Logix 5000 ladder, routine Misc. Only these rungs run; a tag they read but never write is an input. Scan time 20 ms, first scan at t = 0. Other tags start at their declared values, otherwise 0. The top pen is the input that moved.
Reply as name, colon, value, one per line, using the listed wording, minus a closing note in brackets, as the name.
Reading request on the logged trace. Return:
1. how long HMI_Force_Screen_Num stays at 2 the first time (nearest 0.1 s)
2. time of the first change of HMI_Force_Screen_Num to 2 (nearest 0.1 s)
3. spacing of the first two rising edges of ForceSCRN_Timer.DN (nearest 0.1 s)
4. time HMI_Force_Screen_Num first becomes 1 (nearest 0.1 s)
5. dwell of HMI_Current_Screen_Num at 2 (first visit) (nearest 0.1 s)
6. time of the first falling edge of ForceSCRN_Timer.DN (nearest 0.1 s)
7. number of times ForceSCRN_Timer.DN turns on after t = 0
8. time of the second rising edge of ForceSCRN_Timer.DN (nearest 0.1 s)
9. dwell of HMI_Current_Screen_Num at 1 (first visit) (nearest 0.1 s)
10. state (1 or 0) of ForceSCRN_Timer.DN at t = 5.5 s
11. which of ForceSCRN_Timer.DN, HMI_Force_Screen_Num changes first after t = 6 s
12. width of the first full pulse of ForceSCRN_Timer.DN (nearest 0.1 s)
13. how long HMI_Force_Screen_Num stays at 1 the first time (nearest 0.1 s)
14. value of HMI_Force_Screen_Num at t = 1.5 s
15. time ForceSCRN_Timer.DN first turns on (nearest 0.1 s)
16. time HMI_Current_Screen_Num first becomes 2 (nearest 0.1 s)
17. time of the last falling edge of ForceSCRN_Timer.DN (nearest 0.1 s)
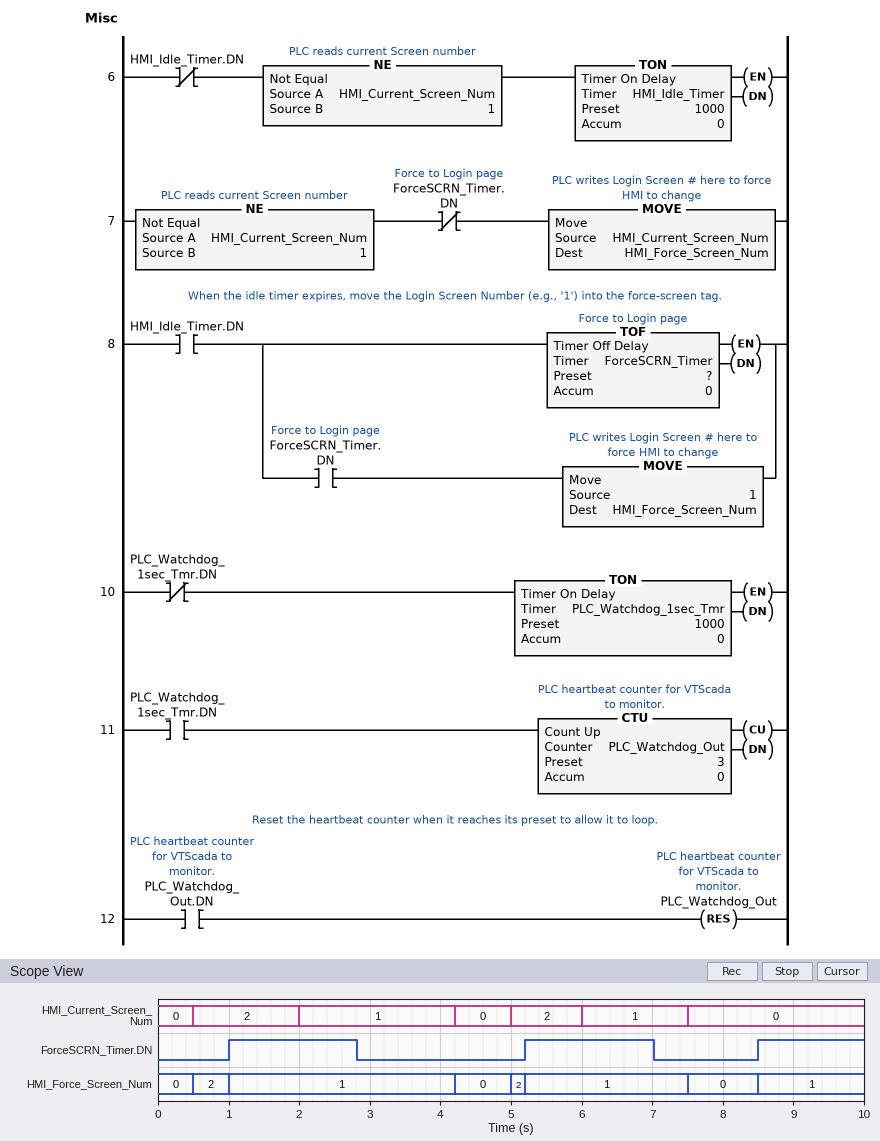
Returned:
how long HMI_Force_Screen_Num stays at 2 the first time: 0.5 s
time of the first change of HMI_Force_Screen_Num to 2: 0.5 s
spacing of the first two rising edges of ForceSCRN_Timer.DN: 4.2 s
time HMI_Force_Screen_Num first becomes 1: 1.0 s
dwell of HMI_Current_Screen_Num at 2 (first visit): 1.5 s
time of the first falling edge of ForceSCRN_Timer.DN: 2.8 s
number of times ForceSCRN_Timer.DN turns on after t = 0: 3
time of the second rising edge of ForceSCRN_Timer.DN: 5.2 s
dwell of HMI_Current_Screen_Num at 1 (first visit): 2.2 s
state (1 or 0) of ForceSCRN_Timer.DN at t = 5.5 s: 1
which of ForceSCRN_Timer.DN, HMI_Force_Screen_Num changes first after t = 6 s: ForceSCRN_Timer.DN
width of the first full pulse of ForceSCRN_Timer.DN: 1.8 s
how long HMI_Force_Screen_Num stays at 1 the first time: 3.2 s
value of HMI_Force_Screen_Num at t = 1.5 s: 1
time ForceSCRN_Timer.DN first turns on: 1.0 s
time HMI_Current_Screen_Num first becomes 2: 0.5 s
time of the last falling edge of ForceSCRN_Timer.DN: 7.0 s
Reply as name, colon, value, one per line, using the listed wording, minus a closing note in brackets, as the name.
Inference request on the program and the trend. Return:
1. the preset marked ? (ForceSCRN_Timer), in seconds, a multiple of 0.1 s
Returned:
the preset marked ? (ForceSCRN_Timer), in seconds, a multiple of 0.1 s: 1.8 s
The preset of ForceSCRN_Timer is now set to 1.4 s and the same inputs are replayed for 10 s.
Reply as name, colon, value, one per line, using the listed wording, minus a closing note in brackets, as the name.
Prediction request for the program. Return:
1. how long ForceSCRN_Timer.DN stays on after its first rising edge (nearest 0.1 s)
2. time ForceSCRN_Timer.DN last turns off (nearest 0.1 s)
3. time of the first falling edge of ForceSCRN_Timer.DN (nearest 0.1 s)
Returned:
how long ForceSCRN_Timer.DN stays on after its first rising edge: 1.4 s
time ForceSCRN_Timer.DN last turns off: 6.6 s
time of the first falling edge of ForceSCRN_Timer.DN: 2.4 s
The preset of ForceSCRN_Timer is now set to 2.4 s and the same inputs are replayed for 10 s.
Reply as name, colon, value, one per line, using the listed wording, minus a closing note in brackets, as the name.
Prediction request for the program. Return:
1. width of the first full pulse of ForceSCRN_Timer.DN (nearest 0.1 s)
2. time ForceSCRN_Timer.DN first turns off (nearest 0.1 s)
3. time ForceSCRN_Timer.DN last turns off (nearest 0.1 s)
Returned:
width of the first full pulse of ForceSCRN_Timer.DN: 2.4 s
time ForceSCRN_Timer.DN first turns off: 3.4 s
time ForceSCRN_Timer.DN last turns off: 7.6 s
